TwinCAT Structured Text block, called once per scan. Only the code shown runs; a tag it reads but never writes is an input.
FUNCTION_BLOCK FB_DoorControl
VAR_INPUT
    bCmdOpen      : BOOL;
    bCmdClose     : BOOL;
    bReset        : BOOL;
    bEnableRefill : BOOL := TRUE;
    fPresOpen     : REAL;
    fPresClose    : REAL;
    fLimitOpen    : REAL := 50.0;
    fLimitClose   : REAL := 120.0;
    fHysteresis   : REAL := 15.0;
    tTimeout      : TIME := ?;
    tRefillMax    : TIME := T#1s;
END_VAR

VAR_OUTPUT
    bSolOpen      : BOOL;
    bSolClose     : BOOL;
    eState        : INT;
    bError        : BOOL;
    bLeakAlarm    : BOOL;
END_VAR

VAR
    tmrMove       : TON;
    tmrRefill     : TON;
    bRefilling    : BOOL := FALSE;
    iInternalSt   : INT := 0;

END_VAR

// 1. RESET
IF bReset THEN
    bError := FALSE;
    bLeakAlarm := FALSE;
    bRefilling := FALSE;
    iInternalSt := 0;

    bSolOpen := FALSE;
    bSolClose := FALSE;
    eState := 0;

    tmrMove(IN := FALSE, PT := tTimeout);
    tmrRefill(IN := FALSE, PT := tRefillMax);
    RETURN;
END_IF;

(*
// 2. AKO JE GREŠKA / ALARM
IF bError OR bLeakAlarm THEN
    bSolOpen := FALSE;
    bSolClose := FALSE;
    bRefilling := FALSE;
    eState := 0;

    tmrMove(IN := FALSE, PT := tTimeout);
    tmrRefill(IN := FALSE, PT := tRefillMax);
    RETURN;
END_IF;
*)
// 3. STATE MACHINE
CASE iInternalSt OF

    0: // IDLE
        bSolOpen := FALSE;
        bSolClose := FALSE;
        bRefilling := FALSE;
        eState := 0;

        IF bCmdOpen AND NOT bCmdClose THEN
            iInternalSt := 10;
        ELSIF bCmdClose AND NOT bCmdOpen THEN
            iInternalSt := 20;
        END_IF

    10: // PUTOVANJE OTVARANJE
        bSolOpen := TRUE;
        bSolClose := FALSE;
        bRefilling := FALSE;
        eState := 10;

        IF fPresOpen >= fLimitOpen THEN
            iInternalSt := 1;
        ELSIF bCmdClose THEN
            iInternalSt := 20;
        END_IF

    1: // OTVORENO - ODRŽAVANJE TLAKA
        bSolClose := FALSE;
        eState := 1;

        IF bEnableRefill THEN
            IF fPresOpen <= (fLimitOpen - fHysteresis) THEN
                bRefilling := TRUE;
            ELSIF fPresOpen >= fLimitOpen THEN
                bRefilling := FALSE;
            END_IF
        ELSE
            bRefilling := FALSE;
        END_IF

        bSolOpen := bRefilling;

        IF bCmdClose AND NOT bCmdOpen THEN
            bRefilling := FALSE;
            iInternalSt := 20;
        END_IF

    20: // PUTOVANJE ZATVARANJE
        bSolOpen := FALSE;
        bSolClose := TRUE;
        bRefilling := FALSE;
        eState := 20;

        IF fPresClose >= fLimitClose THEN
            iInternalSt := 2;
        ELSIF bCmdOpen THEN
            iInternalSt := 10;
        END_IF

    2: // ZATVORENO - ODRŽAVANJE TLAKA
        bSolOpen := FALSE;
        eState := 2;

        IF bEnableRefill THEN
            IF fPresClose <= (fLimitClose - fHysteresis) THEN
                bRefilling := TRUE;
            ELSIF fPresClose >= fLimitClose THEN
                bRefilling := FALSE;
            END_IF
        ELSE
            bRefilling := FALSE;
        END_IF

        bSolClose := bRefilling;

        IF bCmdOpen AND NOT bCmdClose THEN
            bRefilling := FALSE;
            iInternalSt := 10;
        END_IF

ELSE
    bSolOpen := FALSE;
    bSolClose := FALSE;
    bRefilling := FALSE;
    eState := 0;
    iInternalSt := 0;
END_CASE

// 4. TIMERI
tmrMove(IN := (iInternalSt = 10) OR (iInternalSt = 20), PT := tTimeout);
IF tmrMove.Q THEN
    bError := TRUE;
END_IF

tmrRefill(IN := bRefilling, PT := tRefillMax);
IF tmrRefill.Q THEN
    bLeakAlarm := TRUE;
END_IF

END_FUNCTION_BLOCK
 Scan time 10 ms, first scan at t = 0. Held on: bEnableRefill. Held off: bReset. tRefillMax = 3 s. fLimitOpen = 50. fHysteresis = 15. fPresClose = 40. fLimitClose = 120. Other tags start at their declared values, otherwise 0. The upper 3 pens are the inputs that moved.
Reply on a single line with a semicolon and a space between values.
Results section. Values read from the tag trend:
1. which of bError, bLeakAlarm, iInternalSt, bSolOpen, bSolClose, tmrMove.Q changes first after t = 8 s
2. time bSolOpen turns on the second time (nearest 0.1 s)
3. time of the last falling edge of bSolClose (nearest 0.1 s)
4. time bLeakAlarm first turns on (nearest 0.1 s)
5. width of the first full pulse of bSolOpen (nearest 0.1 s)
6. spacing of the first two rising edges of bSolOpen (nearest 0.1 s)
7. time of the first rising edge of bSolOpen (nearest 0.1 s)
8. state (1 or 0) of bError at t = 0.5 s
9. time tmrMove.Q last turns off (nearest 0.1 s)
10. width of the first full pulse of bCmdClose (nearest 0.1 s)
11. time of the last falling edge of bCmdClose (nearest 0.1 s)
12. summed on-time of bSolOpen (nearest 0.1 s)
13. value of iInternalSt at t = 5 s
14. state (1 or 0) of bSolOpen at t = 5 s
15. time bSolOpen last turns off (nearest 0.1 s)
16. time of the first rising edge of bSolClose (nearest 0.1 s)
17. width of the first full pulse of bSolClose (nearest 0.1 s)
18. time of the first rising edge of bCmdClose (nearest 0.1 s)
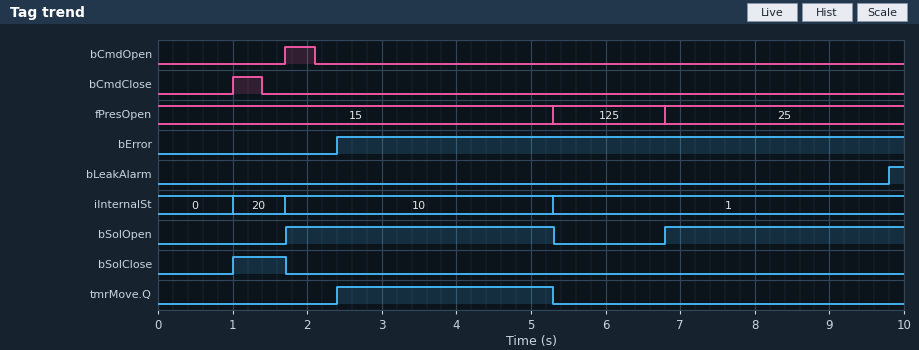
bLeakAlarm; 6.8 s; 1.7 s; 9.8 s; 3.6 s; 5.1 s; 1.7 s; 0; 5.3 s; 0.4 s; 1.4 s; 6.8 s; 10; 1; 5.3 s; 1.0 s; 0.7 s; 1.0 s
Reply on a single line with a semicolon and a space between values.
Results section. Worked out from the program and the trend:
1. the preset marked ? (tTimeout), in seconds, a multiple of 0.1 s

1.4 s
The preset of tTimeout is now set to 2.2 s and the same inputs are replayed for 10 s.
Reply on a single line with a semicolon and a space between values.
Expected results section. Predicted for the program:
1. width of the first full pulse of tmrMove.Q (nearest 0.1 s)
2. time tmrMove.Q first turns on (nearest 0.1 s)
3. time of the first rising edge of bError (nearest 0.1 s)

2.1 s; 3.2 s; 3.2 s
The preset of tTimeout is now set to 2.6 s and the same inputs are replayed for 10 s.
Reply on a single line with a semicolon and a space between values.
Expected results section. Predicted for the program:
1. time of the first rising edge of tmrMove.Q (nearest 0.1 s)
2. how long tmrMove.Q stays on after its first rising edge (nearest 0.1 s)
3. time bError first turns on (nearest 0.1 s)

3.6 s; 1.7 s; 3.6 s
